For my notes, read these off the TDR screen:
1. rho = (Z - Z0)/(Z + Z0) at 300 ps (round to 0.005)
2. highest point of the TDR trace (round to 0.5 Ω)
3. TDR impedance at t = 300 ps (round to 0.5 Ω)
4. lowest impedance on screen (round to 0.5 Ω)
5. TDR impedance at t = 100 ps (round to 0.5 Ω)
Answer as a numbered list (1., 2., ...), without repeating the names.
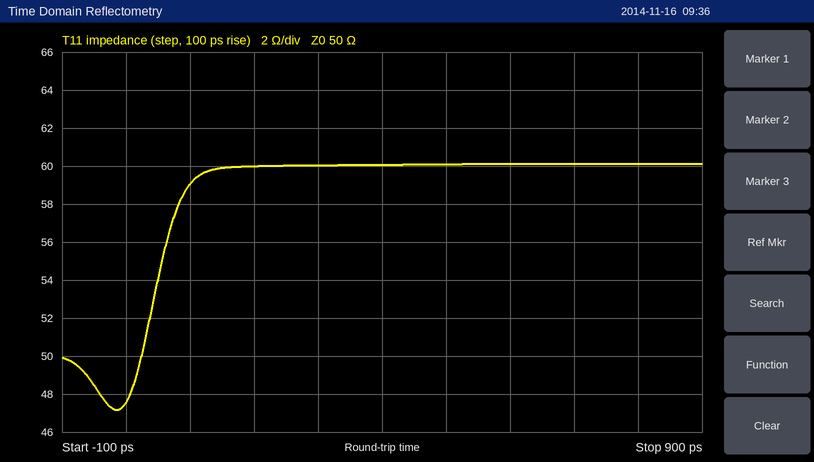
1. +0.090
2. 60.0 Ω
3. 60.0 Ω
4. 47.0 Ω
5. 59.0 Ω
